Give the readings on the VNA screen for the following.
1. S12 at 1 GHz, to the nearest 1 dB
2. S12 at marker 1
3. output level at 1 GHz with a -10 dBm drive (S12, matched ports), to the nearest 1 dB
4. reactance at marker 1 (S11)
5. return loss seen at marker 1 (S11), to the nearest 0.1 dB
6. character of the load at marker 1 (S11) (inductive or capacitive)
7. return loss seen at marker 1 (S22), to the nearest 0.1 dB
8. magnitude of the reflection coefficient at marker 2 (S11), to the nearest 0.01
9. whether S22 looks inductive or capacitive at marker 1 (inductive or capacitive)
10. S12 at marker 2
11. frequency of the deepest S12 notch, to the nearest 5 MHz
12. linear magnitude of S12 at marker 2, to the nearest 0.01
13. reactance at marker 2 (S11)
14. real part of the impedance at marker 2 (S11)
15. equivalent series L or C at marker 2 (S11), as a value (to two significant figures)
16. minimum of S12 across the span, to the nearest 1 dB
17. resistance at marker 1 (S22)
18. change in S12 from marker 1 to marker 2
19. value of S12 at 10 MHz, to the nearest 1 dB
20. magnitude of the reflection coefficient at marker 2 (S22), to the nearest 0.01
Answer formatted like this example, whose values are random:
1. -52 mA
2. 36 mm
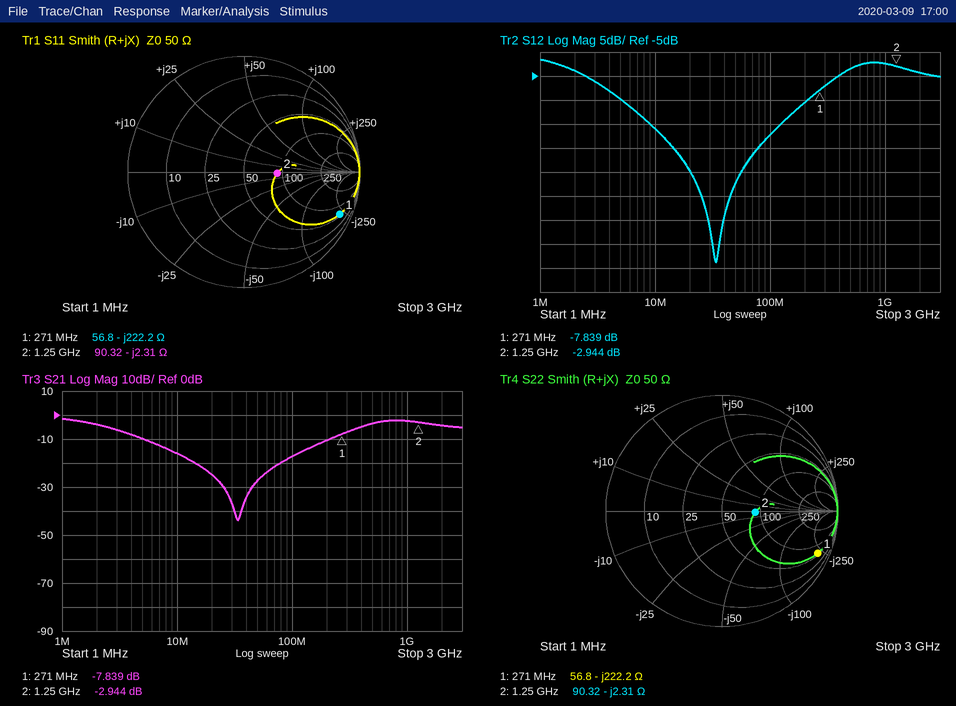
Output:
1. -2 dB
2. -7.839 dB
3. -12 dBm
4. -222.2 Ω
5. 0.9 dB
6. capacitive
7. 0.9 dB
8. 0.29
9. capacitive
10. -2.944 dB
11. 35 MHz
12. 0.71
13. -2.31 Ω
14. 90.32 Ω
15. 55 pF
16. -44 dB
17. 56.8 Ω
18. 4.895 dB
19. -16 dB
20. 0.29
